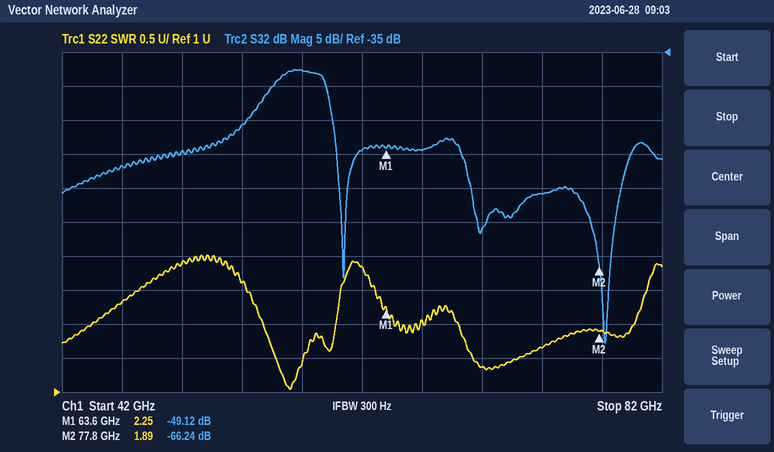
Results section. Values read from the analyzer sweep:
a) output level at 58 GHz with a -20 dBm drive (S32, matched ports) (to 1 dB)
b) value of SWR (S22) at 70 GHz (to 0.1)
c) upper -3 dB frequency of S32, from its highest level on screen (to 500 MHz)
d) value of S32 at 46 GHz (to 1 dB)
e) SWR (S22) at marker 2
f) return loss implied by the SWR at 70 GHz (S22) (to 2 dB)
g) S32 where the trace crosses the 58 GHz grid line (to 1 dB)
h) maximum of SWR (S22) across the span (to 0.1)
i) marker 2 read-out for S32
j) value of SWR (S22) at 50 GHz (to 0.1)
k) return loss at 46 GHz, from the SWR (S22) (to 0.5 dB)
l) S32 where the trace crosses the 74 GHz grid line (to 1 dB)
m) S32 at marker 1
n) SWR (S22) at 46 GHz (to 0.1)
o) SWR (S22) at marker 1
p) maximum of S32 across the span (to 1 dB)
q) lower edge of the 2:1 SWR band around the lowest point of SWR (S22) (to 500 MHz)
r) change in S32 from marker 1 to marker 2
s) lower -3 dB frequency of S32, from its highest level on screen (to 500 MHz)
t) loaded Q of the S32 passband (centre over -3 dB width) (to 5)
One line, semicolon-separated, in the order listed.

-58 dBm; 1.4; 59.5 GHz; -52 dB; 1.89; 16 dB; -38 dB; 3.0; -66.24 dB; 2.9; 8.0 dB; -56 dB; -49.12 dB; 2.3; 2.25; -38 dB; 55.5 GHz; -17.12 dB; 56.0 GHz; 15
